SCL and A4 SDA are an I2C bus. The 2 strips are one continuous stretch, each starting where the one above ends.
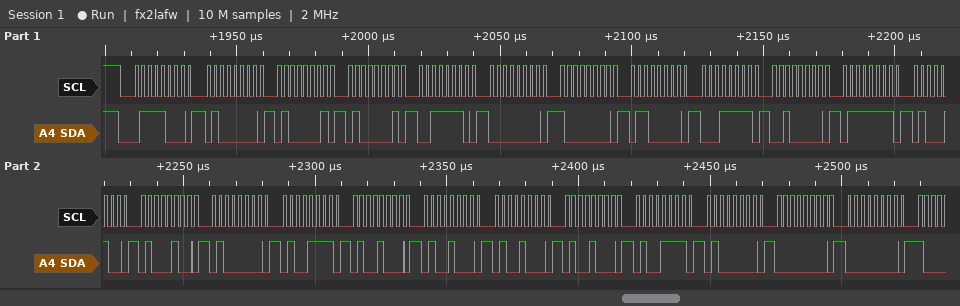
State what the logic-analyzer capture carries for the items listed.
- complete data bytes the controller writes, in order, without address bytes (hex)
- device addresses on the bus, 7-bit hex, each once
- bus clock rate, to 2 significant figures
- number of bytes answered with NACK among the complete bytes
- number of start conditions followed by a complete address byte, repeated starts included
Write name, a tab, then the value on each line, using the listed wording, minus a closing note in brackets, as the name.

complete data bytes the controller writes, in order, without address bytes	40 41 41 3E 00 80 60 1F 20 7F 44 44 40 4F 48 48 48 48 4F 40 00 00
device addresses on the bus, 7-bit hex, each once	0x3C
bus clock rate, to 2 significant figures	400 kHz
number of bytes answered with NACK among the complete bytes	0
number of start conditions followed by a complete address byte, repeated starts included	1
